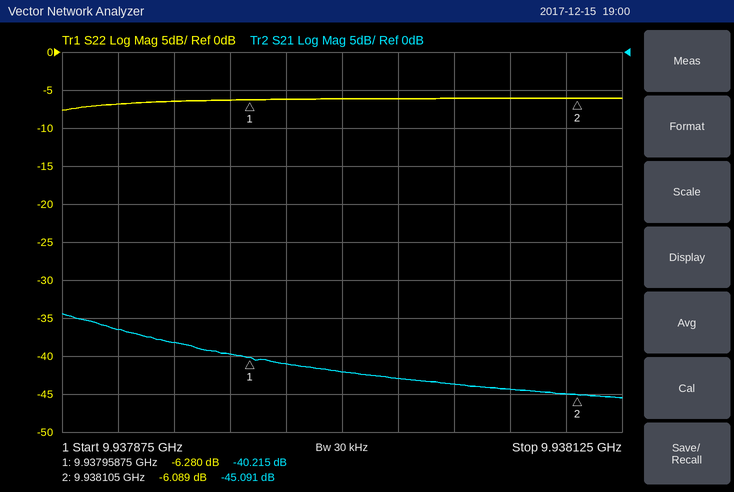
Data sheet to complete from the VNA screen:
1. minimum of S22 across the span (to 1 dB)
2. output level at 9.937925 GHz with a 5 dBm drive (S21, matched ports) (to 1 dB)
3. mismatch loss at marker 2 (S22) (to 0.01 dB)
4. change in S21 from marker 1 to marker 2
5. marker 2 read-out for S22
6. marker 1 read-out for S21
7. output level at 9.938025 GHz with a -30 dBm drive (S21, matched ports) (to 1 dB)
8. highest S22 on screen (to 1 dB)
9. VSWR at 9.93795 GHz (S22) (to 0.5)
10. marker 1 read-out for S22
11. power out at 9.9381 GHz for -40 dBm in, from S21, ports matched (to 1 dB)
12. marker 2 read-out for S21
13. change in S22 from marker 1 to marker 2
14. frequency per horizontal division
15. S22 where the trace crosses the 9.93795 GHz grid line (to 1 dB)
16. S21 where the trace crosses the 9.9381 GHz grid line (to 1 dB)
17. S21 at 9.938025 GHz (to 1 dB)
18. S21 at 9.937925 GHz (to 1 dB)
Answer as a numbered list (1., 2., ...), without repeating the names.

1. -8 dB
2. -33 dBm
3. 1.23 dB
4. -4.876 dB
5. -6.089 dB
6. -40.215 dB
7. -73 dBm
8. -6 dB
9. 3.0
10. -6.280 dB
11. -85 dBm
12. -45.091 dB
13. 0.191 dB
14. 25 kHz
15. -6 dB
16. -45 dB
17. -43 dB
18. -38 dB
